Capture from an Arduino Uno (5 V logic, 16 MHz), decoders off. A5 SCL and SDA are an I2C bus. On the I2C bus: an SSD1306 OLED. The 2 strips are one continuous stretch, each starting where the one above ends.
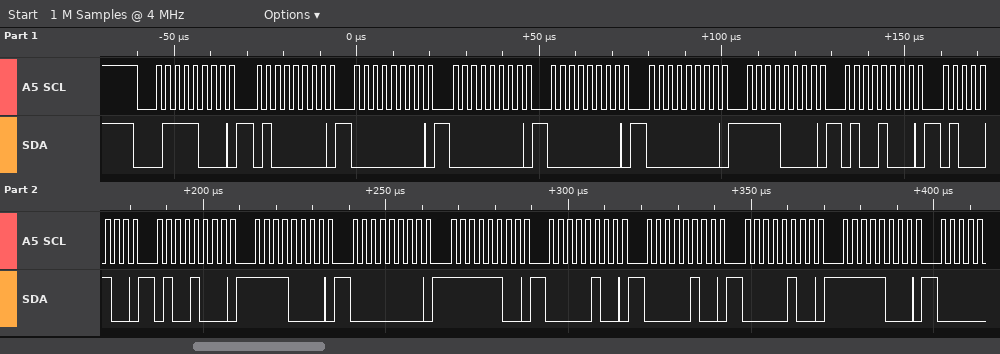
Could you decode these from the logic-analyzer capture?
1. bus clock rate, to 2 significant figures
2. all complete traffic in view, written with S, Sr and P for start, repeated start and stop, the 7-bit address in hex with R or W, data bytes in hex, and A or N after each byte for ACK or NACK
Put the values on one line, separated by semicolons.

400 kHz; S 3CW A 40 A 00 A 00 A 00 A 00 A F0 A 48 A 44 A 48 A F0 A 00 A FC A 04 A 04 A 04 A F8 A
